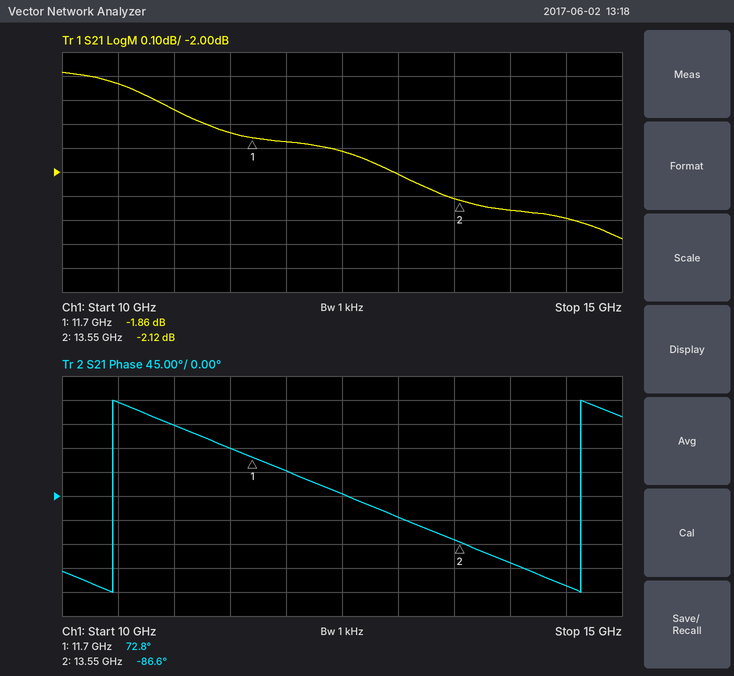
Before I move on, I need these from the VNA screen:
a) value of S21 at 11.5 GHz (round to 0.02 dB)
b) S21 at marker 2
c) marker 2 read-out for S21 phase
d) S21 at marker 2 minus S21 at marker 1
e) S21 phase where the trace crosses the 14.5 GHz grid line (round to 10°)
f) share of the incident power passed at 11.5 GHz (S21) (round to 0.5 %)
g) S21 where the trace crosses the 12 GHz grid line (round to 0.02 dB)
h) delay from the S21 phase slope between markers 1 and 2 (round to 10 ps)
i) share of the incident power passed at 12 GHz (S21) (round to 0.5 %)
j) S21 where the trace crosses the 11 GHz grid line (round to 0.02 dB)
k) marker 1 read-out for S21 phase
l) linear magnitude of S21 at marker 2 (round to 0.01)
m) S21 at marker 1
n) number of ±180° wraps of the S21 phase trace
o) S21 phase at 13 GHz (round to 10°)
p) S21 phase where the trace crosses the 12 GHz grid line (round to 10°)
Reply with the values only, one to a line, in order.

-1.84 dB
-2.12 dB
-86.6°
-0.26 dB
-170°
65.5 %
-1.88 dB
240 ps
65.0 %
-1.74 dB
72.8°
0.78
-1.86 dB
2
-40°
50°
